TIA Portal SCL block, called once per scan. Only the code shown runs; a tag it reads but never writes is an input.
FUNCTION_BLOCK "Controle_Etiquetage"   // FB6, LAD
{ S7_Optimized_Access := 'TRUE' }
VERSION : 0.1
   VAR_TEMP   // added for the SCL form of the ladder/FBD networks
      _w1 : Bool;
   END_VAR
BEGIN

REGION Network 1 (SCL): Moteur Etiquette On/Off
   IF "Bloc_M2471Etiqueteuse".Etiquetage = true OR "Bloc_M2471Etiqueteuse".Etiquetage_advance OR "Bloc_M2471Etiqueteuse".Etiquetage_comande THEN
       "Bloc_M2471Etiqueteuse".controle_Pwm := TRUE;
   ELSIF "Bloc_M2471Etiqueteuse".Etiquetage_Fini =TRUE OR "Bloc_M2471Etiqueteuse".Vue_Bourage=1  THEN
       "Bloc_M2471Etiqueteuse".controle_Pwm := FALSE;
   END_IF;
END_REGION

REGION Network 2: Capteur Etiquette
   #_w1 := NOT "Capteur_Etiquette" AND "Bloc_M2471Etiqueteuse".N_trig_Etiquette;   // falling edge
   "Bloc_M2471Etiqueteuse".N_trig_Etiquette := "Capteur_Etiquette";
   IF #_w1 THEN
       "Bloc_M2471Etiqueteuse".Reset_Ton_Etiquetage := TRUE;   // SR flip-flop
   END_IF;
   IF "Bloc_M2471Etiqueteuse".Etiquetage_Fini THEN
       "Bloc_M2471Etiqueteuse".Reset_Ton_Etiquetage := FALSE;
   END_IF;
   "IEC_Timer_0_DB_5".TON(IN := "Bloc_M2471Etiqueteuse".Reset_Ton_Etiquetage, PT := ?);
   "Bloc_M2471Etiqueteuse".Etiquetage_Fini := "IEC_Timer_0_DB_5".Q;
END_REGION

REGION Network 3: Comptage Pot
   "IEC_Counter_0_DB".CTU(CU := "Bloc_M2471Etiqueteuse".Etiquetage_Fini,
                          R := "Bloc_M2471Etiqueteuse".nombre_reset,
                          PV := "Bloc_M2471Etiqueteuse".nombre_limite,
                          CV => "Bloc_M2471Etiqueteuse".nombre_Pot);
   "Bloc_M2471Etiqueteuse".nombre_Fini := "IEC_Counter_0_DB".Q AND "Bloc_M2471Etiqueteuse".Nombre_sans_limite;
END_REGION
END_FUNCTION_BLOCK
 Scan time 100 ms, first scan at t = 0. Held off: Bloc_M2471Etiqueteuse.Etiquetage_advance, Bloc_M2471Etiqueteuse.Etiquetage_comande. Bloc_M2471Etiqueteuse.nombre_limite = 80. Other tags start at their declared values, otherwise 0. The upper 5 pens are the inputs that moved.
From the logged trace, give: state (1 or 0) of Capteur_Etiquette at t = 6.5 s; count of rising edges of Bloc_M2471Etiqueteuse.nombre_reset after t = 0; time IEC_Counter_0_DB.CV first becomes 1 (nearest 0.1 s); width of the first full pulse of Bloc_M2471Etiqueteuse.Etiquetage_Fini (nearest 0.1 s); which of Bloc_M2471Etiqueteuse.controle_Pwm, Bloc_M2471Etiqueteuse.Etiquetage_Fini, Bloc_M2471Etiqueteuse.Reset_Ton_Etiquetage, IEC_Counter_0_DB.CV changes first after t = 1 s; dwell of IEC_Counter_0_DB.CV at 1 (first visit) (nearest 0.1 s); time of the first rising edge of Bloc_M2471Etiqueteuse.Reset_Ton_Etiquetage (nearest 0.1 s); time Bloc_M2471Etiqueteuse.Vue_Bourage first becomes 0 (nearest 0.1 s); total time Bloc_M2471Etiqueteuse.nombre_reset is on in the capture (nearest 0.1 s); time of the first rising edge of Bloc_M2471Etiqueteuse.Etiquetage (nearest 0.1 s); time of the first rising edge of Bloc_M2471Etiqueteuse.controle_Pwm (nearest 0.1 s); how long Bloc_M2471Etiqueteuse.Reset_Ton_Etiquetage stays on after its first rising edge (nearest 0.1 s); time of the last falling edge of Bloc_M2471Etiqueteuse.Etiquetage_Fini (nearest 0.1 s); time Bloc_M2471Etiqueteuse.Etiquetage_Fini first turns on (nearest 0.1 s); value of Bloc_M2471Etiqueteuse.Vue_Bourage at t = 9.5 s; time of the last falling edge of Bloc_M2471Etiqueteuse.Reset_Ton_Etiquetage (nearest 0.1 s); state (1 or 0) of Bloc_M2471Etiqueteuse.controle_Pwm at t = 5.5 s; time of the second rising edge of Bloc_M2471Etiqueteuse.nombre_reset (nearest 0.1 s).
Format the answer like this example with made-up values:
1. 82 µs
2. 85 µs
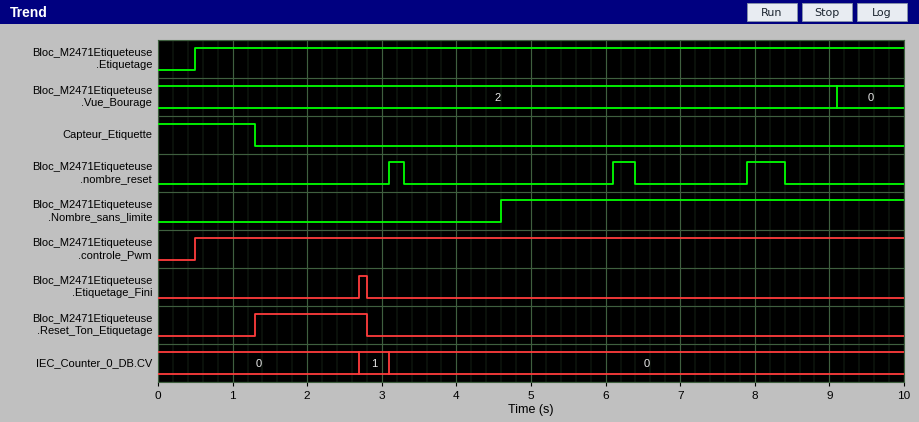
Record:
1. 0
2. 3
3. 2.7 s
4. 0.1 s
5. Bloc_M2471Etiqueteuse.Reset_Ton_Etiquetage
6. 0.4 s
7. 1.3 s
8. 9.1 s
9. 1.0 s
10. 0.5 s
11. 0.5 s
12. 1.5 s
13. 2.8 s
14. 2.7 s
15. 0
16. 2.8 s
17. 1
18. 6.1 s
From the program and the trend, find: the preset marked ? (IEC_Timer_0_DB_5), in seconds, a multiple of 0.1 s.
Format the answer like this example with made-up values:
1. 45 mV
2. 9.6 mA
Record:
1. 1.4 s
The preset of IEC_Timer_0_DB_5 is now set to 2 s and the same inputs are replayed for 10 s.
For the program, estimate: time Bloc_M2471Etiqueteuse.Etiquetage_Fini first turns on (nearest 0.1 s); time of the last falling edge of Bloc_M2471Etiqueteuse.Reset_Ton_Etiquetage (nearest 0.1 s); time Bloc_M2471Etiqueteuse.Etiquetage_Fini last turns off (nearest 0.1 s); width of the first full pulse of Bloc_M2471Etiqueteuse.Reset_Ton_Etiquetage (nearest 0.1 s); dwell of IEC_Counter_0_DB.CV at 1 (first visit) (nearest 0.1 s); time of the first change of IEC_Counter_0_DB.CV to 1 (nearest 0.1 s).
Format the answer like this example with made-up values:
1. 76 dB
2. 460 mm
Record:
1. 3.3 s
2. 3.4 s
3. 3.4 s
4. 2.1 s
5. 2.8 s
6. 3.3 s
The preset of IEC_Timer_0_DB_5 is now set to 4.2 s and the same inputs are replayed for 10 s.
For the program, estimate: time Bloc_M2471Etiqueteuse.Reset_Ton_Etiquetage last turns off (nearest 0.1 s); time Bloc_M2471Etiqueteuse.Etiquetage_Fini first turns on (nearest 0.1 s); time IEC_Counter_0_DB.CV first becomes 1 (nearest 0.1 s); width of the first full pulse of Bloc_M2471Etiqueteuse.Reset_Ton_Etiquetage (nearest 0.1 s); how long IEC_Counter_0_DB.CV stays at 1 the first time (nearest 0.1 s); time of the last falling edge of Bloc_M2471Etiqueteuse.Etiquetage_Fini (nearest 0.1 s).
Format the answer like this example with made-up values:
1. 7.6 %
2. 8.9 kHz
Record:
1. 5.6 s
2. 5.5 s
3. 5.5 s
4. 4.3 s
5. 0.6 s
6. 5.6 s
